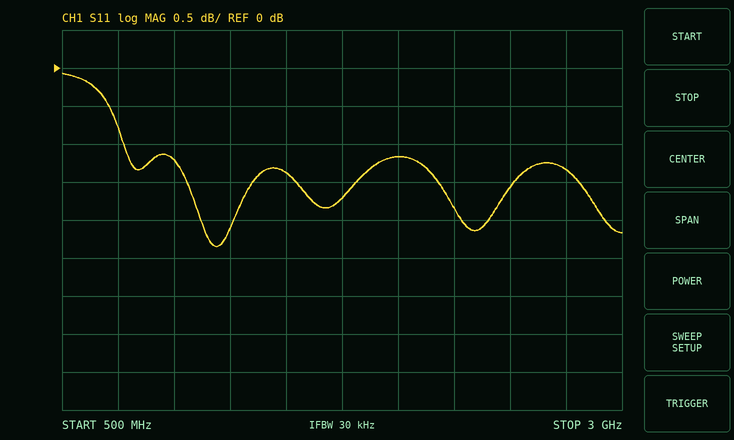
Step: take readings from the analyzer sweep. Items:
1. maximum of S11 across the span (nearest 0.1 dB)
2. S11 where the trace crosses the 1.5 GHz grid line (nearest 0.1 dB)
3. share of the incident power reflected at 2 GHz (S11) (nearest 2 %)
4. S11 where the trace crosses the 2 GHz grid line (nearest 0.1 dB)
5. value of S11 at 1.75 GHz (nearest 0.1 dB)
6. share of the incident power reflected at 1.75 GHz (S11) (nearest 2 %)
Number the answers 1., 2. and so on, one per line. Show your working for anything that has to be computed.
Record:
1. -0.1 dB
2. -1.4 dB
3. 10^(-1.2/10) ≈ 76 %
4. -1.2 dB
5. -1.7 dB
6. 10^(-1.7/10) ≈ 68 %
